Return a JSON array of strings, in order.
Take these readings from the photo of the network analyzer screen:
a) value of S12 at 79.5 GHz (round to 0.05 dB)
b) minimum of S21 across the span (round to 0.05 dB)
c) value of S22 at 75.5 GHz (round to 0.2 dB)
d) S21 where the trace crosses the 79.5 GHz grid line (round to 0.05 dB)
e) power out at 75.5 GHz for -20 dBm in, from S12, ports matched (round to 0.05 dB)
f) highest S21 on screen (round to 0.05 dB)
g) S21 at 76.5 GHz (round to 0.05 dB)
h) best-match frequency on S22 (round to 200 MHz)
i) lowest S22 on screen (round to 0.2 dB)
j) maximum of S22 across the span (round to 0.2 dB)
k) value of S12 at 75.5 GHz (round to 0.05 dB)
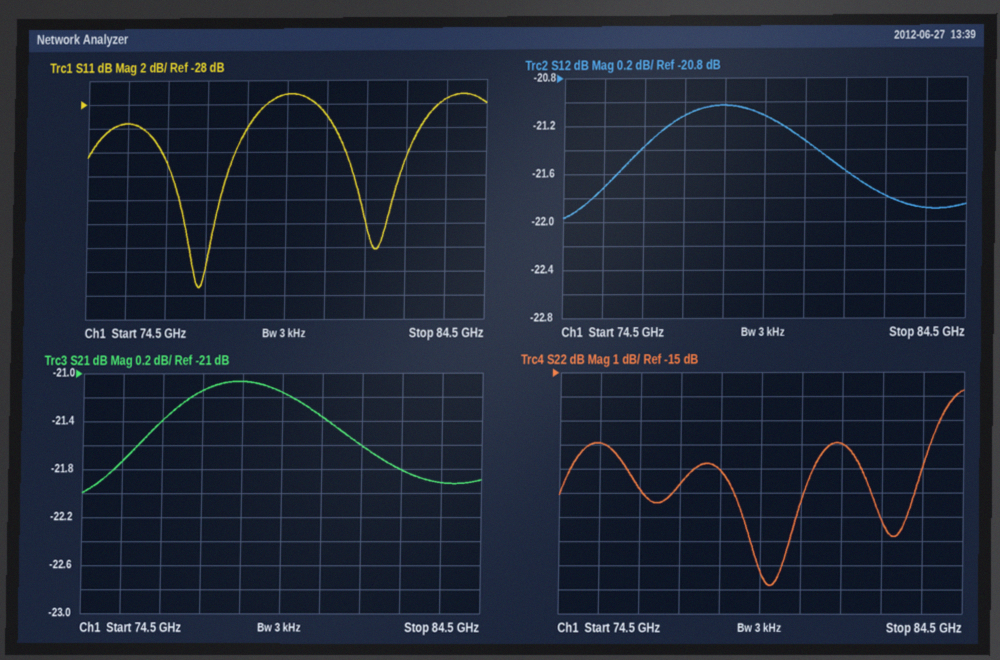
["-21.10 dB", "-22.00 dB", "-18.0 dB", "-21.15 dB", "-41.70 dBm", "-21.05 dB", "-21.40 dB", "79.8 GHz", "-23.8 dB", "-15.8 dB", "-21.70 dB"]
